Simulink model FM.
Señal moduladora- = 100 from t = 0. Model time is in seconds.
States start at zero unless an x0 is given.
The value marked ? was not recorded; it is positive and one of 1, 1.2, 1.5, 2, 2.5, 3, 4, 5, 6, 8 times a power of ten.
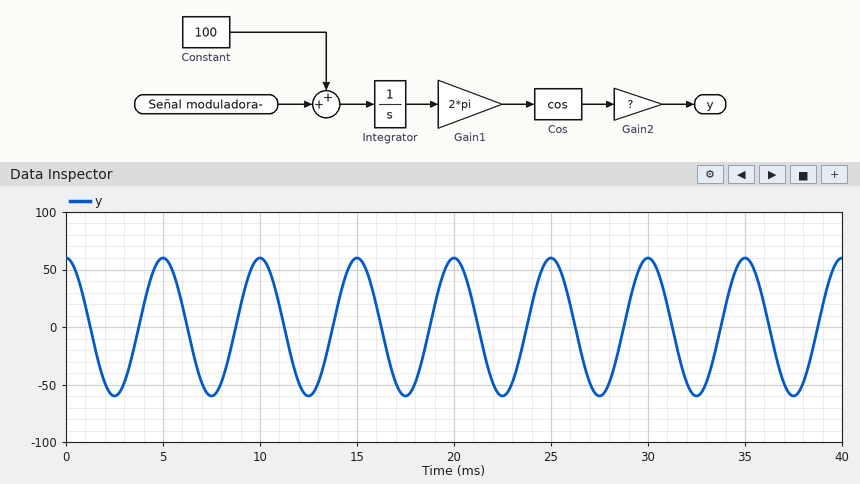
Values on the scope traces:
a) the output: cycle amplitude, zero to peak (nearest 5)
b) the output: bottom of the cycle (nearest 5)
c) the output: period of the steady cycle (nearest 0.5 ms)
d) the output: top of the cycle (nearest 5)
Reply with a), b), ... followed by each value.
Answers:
a) 60
b) -60
c) 5.0 ms
d) 60
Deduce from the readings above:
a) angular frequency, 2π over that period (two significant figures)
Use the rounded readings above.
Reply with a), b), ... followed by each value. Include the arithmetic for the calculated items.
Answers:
a) 2π / 5 = 1.3 rad/ms
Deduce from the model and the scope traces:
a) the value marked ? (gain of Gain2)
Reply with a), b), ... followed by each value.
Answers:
a) 60
